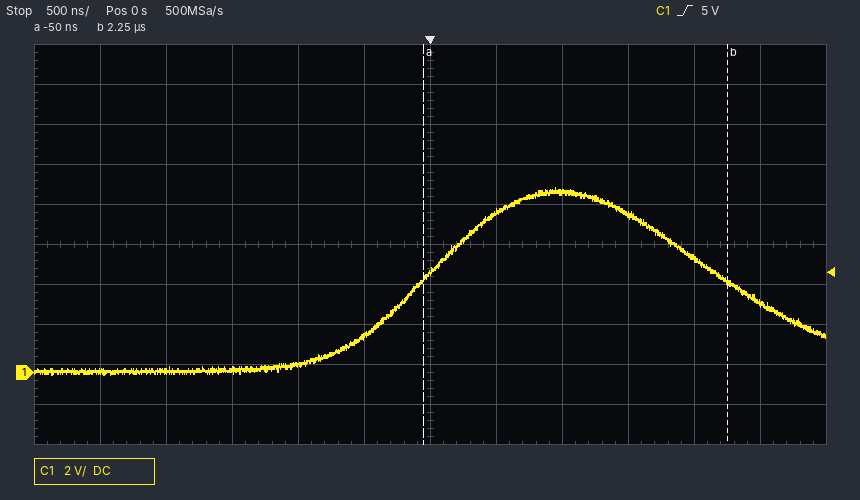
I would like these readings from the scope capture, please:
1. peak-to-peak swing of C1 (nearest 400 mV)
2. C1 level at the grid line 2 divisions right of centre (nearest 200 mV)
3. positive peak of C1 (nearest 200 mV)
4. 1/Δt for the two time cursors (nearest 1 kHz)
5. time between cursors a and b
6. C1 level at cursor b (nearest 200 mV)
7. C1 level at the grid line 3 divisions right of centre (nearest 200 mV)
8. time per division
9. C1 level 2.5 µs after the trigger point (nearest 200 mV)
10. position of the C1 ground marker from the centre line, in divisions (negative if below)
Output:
9.2 V
9.0 V
9.2 V
435 kHz
2.30 µs
4.6 V
7.8 V
500 ns
3.4 V
-3.2 div
